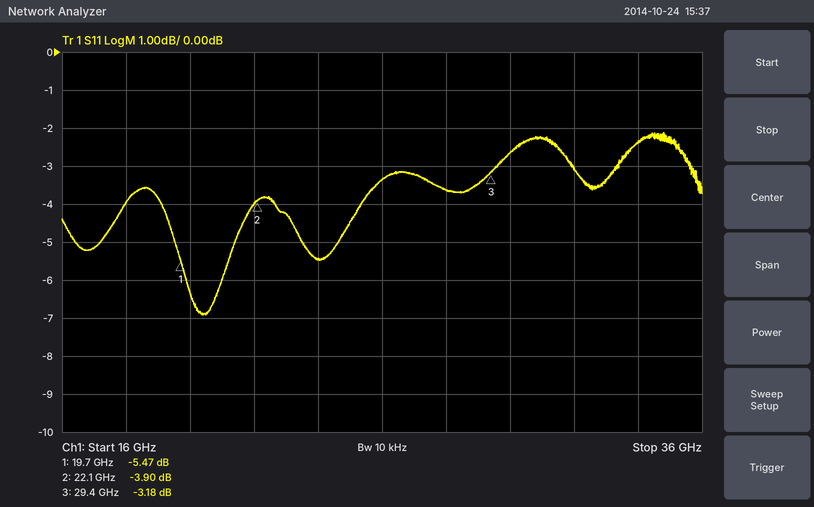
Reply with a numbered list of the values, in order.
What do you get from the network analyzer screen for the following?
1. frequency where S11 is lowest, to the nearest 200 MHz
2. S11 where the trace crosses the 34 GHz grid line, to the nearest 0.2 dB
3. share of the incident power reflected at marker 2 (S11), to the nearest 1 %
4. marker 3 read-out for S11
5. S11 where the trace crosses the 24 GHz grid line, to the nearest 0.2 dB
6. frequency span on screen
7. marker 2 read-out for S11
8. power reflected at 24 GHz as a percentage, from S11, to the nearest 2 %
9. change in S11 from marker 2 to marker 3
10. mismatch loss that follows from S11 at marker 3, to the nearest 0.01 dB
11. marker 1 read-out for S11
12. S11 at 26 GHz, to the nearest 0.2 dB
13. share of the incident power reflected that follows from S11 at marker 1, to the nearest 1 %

1. 20.4 GHz
2. -2.4 dB
3. 41 %
4. -3.18 dB
5. -5.4 dB
6. 20 GHz
7. -3.90 dB
8. 28 %
9. 0.72 dB
10. 2.85 dB
11. -5.47 dB
12. -3.4 dB
13. 28 %
